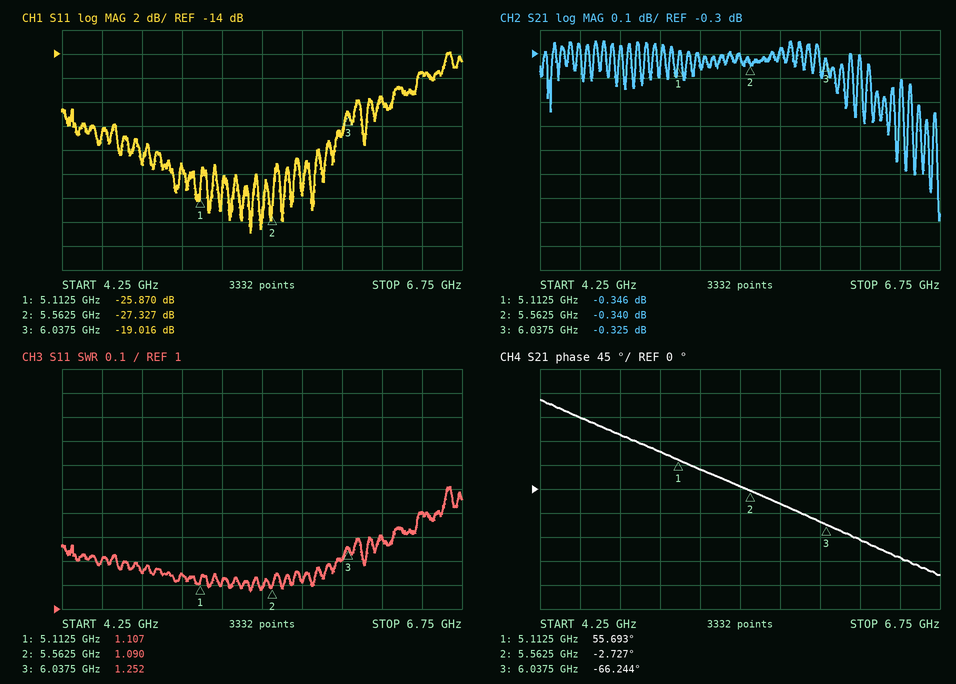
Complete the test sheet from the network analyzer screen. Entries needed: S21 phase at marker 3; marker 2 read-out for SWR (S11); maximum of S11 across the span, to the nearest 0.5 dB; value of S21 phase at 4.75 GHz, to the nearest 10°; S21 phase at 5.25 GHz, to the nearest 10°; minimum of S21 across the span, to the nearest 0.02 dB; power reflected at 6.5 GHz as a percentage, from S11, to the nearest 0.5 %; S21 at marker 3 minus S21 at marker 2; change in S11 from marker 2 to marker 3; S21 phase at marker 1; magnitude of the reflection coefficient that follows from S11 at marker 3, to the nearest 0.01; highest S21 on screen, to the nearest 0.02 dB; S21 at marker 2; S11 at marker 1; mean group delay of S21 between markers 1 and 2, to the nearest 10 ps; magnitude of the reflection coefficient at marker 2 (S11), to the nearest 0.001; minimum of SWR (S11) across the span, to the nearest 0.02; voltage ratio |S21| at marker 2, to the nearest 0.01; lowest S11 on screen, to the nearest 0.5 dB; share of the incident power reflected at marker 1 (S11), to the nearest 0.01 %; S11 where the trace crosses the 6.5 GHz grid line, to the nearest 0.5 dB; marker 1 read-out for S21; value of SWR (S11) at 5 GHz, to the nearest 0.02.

-66.244°
1.090
-14.0 dB
100°
40°
-1.00 dB
3.0 %
0.015 dB
8.311 dB
55.693°
0.11
-0.24 dB
-0.340 dB
-25.870 dB
360 ps
0.043
1.08
0.96
-29.0 dB
0.26 %
-15.5 dB
-0.346 dB
1.14
